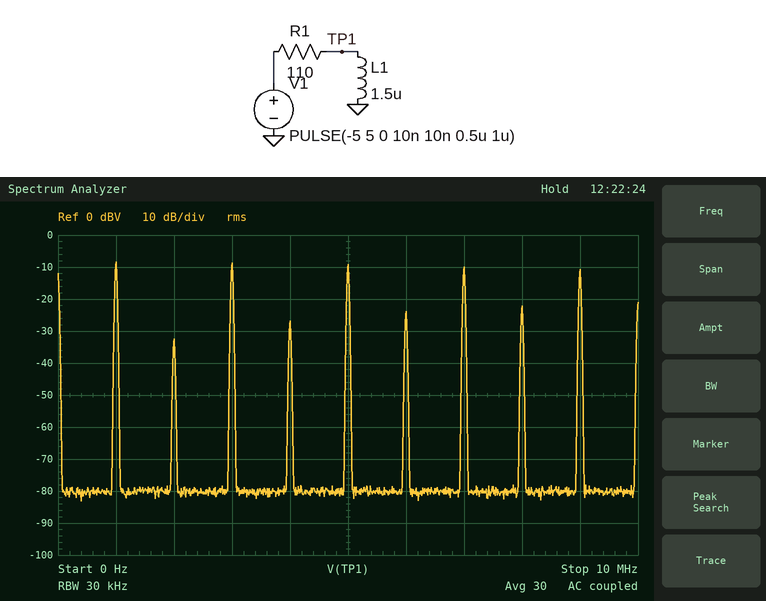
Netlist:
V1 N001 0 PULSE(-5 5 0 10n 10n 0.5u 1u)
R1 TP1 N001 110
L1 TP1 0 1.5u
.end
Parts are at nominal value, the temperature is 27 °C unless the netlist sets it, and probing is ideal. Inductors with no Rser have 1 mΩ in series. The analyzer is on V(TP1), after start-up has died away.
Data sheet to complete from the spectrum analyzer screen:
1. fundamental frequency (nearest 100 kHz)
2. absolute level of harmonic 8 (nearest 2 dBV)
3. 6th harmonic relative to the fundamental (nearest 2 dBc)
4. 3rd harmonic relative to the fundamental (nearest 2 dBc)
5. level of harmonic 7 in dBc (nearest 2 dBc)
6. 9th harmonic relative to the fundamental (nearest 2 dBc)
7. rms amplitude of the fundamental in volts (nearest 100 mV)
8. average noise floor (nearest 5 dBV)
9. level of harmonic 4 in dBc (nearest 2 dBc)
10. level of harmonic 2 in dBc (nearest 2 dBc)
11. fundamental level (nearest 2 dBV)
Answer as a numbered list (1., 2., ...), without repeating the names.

1. 1.0 MHz
2. -22 dBV
3. -16 dBc
4. 0 dBc
5. -2 dBc
6. -2 dBc
7. 400 mV
8. -80 dBV
9. -18 dBc
10. -24 dBc
11. -8 dBV
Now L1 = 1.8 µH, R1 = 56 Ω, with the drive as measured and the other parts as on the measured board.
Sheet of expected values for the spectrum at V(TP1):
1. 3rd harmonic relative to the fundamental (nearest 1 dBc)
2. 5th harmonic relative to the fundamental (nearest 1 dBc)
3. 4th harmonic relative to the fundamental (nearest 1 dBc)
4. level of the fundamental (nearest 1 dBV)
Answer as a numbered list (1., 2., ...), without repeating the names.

1. -1 dBc
2. -3 dBc
3. -20 dBc
4. -1 dBV
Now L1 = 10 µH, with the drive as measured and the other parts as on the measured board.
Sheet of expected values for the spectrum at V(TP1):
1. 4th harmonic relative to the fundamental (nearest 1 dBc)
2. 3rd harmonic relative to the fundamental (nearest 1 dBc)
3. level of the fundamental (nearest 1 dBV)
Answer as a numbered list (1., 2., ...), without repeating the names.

1. -25 dBc
2. -5 dBc
3. 7 dBV
